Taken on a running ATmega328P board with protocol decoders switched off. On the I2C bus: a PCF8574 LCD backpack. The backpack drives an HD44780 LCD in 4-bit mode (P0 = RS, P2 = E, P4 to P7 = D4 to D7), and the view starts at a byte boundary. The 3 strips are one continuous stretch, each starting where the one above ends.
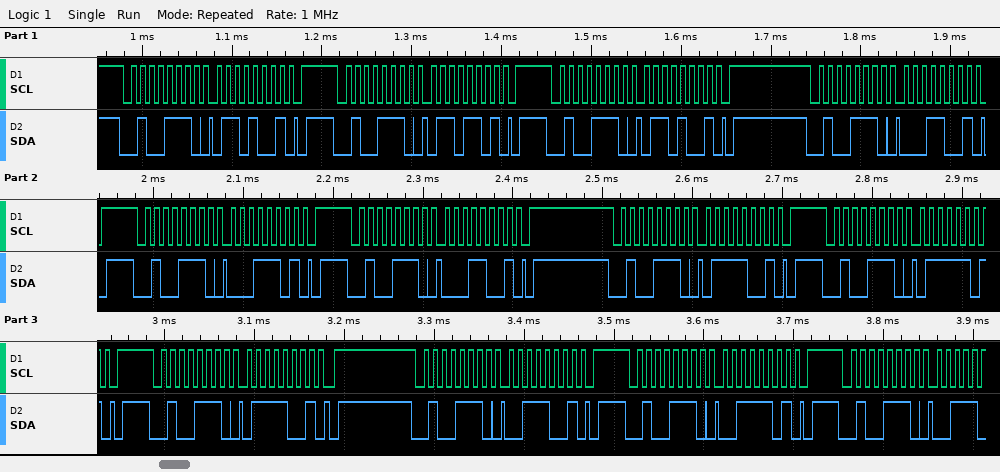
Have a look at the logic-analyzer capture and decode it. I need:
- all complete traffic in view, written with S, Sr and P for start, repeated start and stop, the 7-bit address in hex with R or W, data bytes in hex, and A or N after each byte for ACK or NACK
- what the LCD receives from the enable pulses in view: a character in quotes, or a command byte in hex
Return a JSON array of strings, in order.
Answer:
["S 27W A 69 A P S 27W A 6D A P S 27W A 69 A P S 27W A 19 A P S 27W A 1D A P S 27W A 19 A P S 27W A 79 A P S 27W A 7D A P S 27W A 79 A P S 27W A 39 A P S 27W A 3D A P S 27W A", "'a'"]
